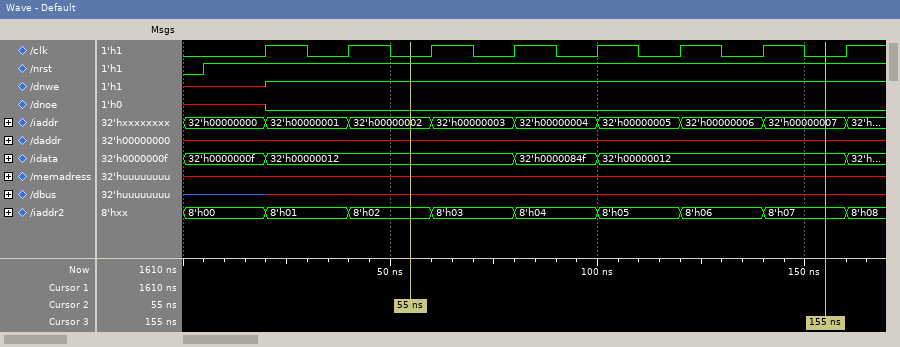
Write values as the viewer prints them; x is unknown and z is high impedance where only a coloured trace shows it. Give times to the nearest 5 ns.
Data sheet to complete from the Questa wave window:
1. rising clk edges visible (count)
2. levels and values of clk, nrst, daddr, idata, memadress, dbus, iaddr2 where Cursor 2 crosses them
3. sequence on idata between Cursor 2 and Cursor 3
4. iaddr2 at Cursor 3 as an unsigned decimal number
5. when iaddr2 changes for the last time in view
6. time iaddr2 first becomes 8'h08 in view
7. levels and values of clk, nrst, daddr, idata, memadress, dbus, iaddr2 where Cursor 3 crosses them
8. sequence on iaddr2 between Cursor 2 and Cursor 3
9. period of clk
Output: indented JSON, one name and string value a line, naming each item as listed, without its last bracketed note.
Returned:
{
  "rising clk edges visible": "8",
  "levels and values of clk, nrst, daddr, idata, memadress, dbus, iaddr2 where Cursor 2 crosses them": "clk=0, nrst=1, daddr=x, idata=32'h00000012, memadress=x, dbus=x, iaddr2=8'h02",
  "sequence on idata between Cursor 2 and Cursor 3": "32'h00000012, 32'h0000084f, 32'h00000012",
  "iaddr2 at Cursor 3 as an unsigned decimal number": "7",
  "when iaddr2 changes for the last time in view": "160 ns",
  "time iaddr2 first becomes 8'h08 in view": "160 ns",
  "levels and values of clk, nrst, daddr, idata, memadress, dbus, iaddr2 where Cursor 3 crosses them": "clk=0, nrst=1, daddr=x, idata=32'h00000012, memadress=x, dbus=x, iaddr2=8'h07",
  "sequence on iaddr2 between Cursor 2 and Cursor 3": "8'h02, 8'h03, 8'h04, 8'h05, 8'h06, 8'h07",
  "period of clk": "20 ns"
}
